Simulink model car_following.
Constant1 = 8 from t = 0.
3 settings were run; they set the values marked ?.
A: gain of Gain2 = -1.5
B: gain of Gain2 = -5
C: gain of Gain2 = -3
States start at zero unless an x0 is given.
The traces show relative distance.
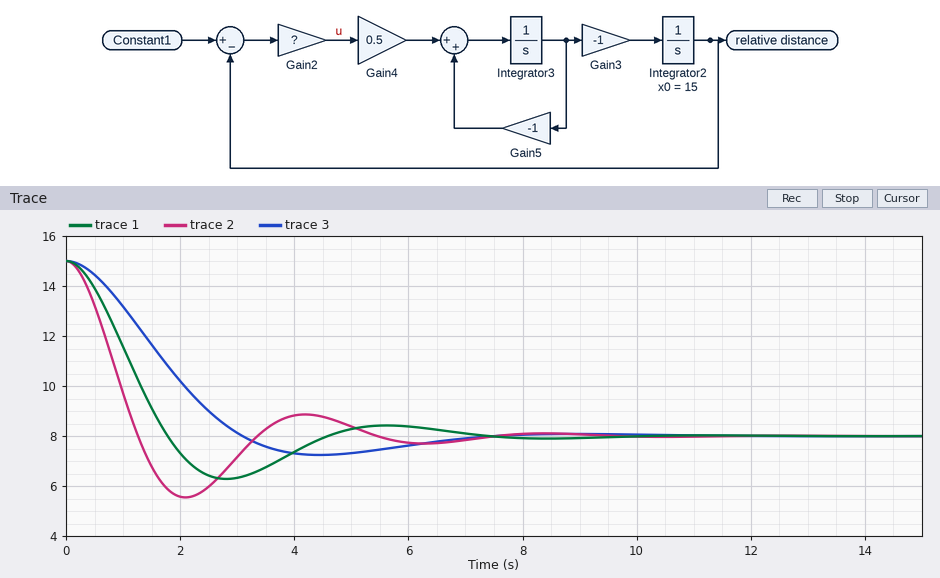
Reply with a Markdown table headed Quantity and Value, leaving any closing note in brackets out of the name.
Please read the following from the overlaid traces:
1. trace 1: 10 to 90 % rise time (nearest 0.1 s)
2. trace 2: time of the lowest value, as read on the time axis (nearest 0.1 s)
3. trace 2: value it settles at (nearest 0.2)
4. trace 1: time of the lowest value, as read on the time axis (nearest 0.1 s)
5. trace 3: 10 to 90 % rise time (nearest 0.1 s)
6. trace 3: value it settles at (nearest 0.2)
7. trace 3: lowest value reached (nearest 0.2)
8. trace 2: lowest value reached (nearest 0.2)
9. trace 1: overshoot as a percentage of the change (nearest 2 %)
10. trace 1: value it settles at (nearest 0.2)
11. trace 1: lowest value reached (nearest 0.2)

| Quantity | Value |
|---|---|
| trace 1: 10 to 90 % rise time | 1.2 s |
| trace 2: time of the lowest value, as read on the time axis | 2.1 s |
| trace 2: value it settles at | 8.0 |
| trace 1: time of the lowest value, as read on the time axis | 2.8 s |
| trace 3: 10 to 90 % rise time | 2.1 s |
| trace 3: value it settles at | 8.0 |
| trace 3: lowest value reached | 7.2 |
| trace 2: lowest value reached | 5.6 |
| trace 1: overshoot as a percentage of the change | 24 % |
| trace 1: value it settles at | 8.0 |
| trace 1: lowest value reached | 6.2 |
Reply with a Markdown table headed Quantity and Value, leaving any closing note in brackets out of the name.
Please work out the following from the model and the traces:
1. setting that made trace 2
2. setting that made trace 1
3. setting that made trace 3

| Quantity | Value |
|---|---|
| setting that made trace 2 | B |
| setting that made trace 1 | C |
| setting that made trace 3 | A |
